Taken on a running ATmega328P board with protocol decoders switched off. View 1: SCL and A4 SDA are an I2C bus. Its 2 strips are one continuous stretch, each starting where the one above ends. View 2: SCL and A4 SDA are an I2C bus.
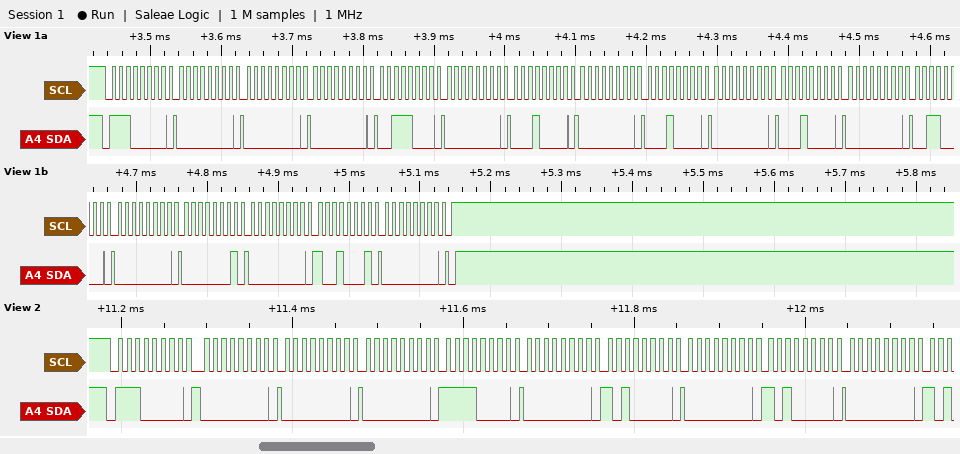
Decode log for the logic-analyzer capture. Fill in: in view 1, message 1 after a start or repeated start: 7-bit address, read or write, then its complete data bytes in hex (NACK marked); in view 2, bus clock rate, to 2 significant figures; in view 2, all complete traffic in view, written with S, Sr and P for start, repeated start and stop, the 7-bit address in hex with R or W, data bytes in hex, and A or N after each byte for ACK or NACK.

0x70 write: 00 00 00 38 00 10 00 10 00 10 00 30 00 01 00 91 00
100 kHz
S 70W A 00 A 00 A 00 A F0 A 00 A A0 A 00 A A0 A 00 A
